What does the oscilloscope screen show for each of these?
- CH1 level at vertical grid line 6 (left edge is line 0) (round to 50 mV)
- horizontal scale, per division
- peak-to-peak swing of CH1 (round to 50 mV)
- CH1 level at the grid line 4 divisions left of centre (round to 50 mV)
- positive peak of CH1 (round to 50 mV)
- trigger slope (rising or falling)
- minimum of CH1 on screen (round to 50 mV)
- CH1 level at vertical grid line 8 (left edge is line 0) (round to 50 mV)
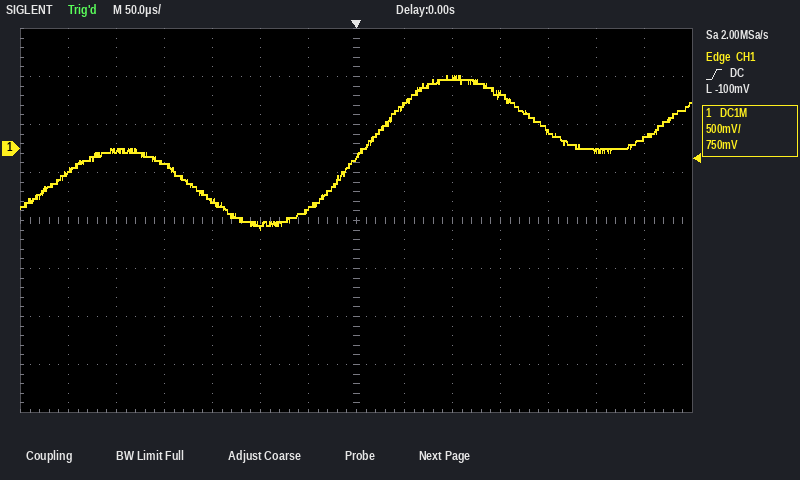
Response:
-650 mV
50 µs
1.60 V
-150 mV
750 mV
rising
-850 mV
450 mV
